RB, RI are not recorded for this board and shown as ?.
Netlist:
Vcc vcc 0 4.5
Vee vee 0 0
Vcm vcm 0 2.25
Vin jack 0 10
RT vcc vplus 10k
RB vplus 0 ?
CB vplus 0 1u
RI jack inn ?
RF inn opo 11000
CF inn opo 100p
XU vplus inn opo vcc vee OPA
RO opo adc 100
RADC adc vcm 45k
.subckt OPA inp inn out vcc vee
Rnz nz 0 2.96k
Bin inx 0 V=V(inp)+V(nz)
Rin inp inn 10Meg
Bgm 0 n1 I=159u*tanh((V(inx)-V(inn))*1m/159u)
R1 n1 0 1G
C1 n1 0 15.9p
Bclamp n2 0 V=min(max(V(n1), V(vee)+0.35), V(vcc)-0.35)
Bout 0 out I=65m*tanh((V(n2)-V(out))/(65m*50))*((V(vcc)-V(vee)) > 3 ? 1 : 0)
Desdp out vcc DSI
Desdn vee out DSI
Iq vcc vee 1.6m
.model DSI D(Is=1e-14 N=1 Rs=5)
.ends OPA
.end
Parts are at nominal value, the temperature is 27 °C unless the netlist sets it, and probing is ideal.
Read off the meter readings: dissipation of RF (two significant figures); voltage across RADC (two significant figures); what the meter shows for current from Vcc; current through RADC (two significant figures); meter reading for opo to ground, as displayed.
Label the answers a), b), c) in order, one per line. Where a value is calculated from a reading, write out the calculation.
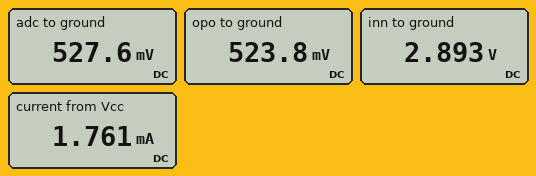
a) (2.893 V - 523.8 mV)^2 / 11 kΩ = 510 µW
b) 2.25 V - 527.6 mV = 1.7 V
c) 1.761 mA
d) (2.25 V - 527.6 mV) / 45 kΩ = 38 µA
e) 523.8 mV
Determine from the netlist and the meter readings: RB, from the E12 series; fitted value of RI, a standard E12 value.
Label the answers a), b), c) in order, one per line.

a) 18 kΩ
b) 33 kΩ
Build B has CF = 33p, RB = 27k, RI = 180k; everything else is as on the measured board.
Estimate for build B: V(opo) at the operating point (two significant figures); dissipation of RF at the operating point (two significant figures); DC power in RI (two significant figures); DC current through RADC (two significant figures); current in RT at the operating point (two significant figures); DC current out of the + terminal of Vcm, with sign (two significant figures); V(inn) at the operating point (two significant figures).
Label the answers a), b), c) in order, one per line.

a) 2.9 V
b) 15 µW
c) 250 µW
d) 14 µA
e) 120 µA
f) -14 µA
g) 3.3 V
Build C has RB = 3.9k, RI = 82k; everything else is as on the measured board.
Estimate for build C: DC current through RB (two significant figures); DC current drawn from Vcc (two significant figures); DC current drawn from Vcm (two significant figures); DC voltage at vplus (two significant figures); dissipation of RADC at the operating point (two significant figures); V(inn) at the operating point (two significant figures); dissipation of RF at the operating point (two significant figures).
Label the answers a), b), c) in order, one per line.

a) 320 µA
b) 1.9 mA
c) 42 µA
d) 1.3 V
e) 79 µW
f) 1.5 V
g) 120 µW
